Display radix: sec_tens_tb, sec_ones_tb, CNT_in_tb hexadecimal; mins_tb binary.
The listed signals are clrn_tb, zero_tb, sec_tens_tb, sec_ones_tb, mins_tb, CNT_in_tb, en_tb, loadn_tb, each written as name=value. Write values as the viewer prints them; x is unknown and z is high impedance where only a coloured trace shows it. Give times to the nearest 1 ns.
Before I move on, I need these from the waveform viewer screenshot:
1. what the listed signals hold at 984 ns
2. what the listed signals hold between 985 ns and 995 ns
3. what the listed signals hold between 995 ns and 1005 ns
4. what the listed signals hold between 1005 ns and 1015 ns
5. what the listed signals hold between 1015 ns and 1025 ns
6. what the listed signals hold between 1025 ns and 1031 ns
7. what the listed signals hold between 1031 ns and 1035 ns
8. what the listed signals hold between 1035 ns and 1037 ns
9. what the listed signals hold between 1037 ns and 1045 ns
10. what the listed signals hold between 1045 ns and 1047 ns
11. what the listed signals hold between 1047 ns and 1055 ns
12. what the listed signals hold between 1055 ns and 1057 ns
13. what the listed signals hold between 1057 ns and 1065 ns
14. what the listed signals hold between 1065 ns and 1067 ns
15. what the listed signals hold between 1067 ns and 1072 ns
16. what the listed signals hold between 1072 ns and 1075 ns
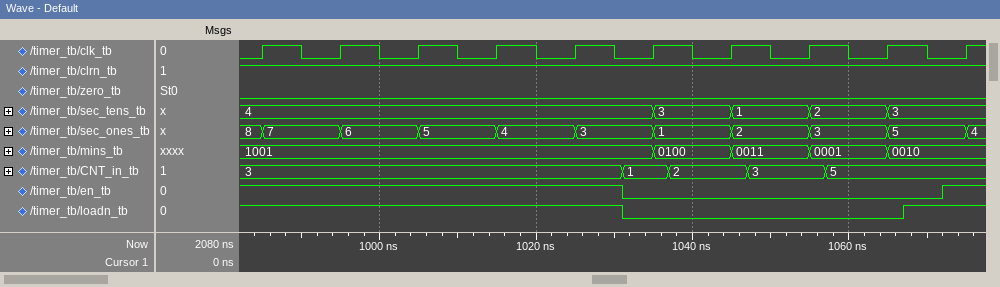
clrn_tb=1, zero_tb=0, sec_tens_tb=4, sec_ones_tb=8, mins_tb=1001, CNT_in_tb=3, en_tb=1, loadn_tb=1
clrn_tb=1, zero_tb=0, sec_tens_tb=4, sec_ones_tb=7, mins_tb=1001, CNT_in_tb=3, en_tb=1, loadn_tb=1
clrn_tb=1, zero_tb=0, sec_tens_tb=4, sec_ones_tb=6, mins_tb=1001, CNT_in_tb=3, en_tb=1, loadn_tb=1
clrn_tb=1, zero_tb=0, sec_tens_tb=4, sec_ones_tb=5, mins_tb=1001, CNT_in_tb=3, en_tb=1, loadn_tb=1
clrn_tb=1, zero_tb=0, sec_tens_tb=4, sec_ones_tb=4, mins_tb=1001, CNT_in_tb=3, en_tb=1, loadn_tb=1
clrn_tb=1, zero_tb=0, sec_tens_tb=4, sec_ones_tb=3, mins_tb=1001, CNT_in_tb=3, en_tb=1, loadn_tb=1
clrn_tb=1, zero_tb=0, sec_tens_tb=4, sec_ones_tb=3, mins_tb=1001, CNT_in_tb=1, en_tb=0, loadn_tb=0
clrn_tb=1, zero_tb=0, sec_tens_tb=3, sec_ones_tb=1, mins_tb=0100, CNT_in_tb=1, en_tb=0, loadn_tb=0
clrn_tb=1, zero_tb=0, sec_tens_tb=3, sec_ones_tb=1, mins_tb=0100, CNT_in_tb=2, en_tb=0, loadn_tb=0
clrn_tb=1, zero_tb=0, sec_tens_tb=1, sec_ones_tb=2, mins_tb=0011, CNT_in_tb=2, en_tb=0, loadn_tb=0
clrn_tb=1, zero_tb=0, sec_tens_tb=1, sec_ones_tb=2, mins_tb=0011, CNT_in_tb=3, en_tb=0, loadn_tb=0
clrn_tb=1, zero_tb=0, sec_tens_tb=2, sec_ones_tb=3, mins_tb=0001, CNT_in_tb=3, en_tb=0, loadn_tb=0
clrn_tb=1, zero_tb=0, sec_tens_tb=2, sec_ones_tb=3, mins_tb=0001, CNT_in_tb=5, en_tb=0, loadn_tb=0
clrn_tb=1, zero_tb=0, sec_tens_tb=3, sec_ones_tb=5, mins_tb=0010, CNT_in_tb=5, en_tb=0, loadn_tb=0
clrn_tb=1, zero_tb=0, sec_tens_tb=3, sec_ones_tb=5, mins_tb=0010, CNT_in_tb=5, en_tb=0, loadn_tb=1
clrn_tb=1, zero_tb=0, sec_tens_tb=3, sec_ones_tb=5, mins_tb=0010, CNT_in_tb=5, en_tb=1, loadn_tb=1
